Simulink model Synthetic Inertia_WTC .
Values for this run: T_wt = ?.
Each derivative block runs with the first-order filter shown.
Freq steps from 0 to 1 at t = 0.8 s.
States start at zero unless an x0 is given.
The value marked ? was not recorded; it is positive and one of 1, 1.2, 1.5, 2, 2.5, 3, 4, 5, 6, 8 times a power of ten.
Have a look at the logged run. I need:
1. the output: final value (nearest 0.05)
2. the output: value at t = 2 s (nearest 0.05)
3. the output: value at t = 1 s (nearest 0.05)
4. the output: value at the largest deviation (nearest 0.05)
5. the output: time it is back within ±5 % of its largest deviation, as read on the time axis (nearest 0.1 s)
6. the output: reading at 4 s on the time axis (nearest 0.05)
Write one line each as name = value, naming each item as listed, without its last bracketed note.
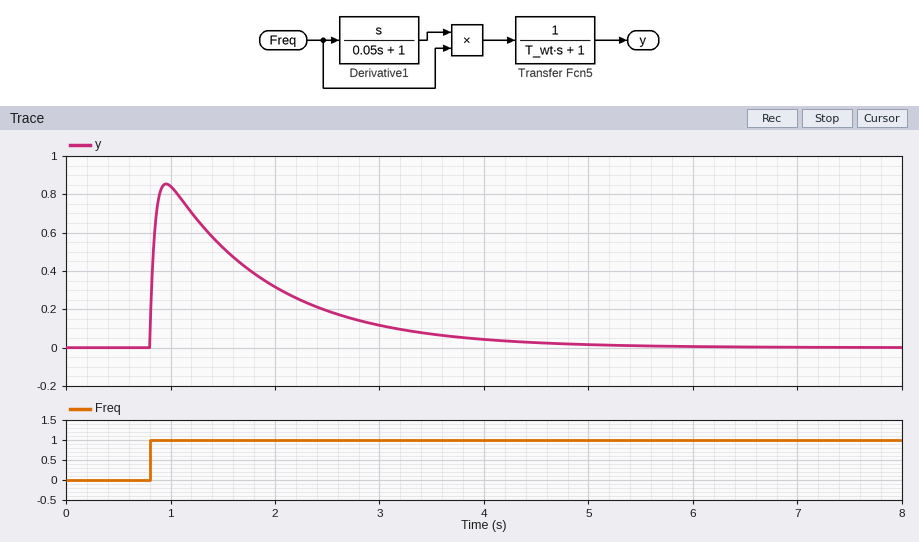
the output: final value = 0.00
the output: value at t = 2 s = 0.30
the output: value at t = 1 s = 0.85
the output: value at the largest deviation = 0.85
the output: time it is back within ±5 % of its largest deviation, as read on the time axis = 4.0 s
the output: reading at 4 s on the time axis = 0.05
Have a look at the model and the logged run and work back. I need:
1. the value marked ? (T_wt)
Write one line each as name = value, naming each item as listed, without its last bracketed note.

the value marked ? = 1
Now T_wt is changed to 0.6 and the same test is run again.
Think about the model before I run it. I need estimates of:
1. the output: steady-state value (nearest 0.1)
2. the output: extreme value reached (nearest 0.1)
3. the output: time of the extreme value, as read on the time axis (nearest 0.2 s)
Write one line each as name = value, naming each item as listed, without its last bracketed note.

the output: steady-state value = 0.0
the output: extreme value reached = 1.3
the output: time of the extreme value, as read on the time axis = 1.0 s
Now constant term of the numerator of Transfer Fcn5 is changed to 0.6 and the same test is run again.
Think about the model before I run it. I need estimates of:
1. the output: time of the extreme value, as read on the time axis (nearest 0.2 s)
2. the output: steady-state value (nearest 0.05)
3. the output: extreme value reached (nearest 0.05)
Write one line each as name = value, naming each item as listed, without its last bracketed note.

the output: time of the extreme value, as read on the time axis = 1.0 s
the output: steady-state value = 0.00
the output: extreme value reached = 0.50
